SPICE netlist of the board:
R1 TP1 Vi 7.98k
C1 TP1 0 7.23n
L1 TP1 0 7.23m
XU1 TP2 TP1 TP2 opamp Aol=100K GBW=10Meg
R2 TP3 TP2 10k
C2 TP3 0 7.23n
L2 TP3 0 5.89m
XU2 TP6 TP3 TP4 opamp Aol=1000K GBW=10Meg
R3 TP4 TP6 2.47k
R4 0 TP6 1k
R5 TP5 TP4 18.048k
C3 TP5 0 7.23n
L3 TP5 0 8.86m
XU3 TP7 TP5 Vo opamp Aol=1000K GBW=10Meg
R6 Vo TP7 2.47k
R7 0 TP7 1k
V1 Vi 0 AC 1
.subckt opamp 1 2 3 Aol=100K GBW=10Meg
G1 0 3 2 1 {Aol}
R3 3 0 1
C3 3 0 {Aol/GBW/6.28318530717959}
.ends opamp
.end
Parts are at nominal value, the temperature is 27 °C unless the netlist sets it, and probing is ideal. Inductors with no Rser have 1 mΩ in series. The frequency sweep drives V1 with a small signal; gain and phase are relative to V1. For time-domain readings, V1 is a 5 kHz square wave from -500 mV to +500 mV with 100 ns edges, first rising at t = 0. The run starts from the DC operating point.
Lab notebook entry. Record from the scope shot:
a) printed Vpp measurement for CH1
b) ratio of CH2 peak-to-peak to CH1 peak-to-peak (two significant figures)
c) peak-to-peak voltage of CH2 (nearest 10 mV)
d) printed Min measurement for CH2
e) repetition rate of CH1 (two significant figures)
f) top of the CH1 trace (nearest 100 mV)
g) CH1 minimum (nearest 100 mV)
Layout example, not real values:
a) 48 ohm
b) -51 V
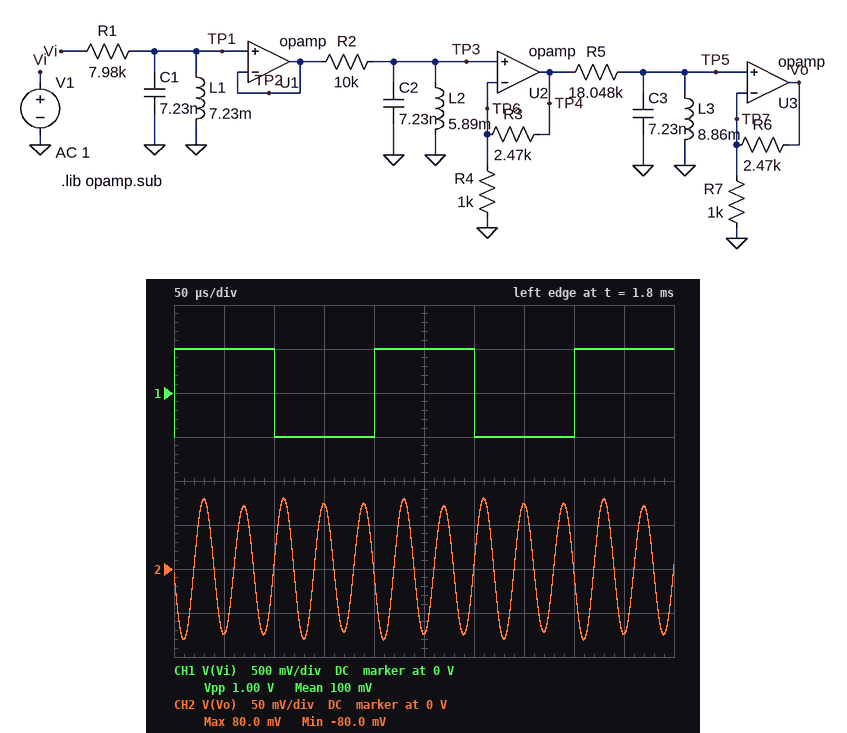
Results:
a) 1.00 V
b) 0.16
c) 160 mV
d) -80.0 mV
e) 5.0 kHz
f) 500 mV
g) -500 mV
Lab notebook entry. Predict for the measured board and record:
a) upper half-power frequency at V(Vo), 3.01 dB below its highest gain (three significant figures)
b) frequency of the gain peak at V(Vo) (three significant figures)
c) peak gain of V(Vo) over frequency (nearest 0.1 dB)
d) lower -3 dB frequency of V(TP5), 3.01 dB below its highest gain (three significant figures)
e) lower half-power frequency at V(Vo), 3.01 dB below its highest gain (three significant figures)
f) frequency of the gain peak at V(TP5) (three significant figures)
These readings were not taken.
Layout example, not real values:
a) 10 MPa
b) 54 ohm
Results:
a) 24.1 kHz
b) 20.2 kHz
c) 3.3 dB
d) 19.6 kHz
e) 19.6 kHz
f) 20.2 kHz
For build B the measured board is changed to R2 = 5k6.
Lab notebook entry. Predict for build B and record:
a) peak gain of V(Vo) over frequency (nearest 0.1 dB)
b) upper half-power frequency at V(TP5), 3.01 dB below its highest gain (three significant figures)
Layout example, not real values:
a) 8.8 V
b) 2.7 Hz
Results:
a) 7.9 dB
b) 22.8 kHz
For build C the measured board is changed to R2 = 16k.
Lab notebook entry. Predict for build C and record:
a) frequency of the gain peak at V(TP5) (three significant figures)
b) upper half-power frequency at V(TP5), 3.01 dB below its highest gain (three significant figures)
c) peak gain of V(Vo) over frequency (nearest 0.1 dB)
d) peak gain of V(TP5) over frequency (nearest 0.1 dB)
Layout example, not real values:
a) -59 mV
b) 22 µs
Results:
a) 24.1 kHz
b) 24.7 kHz
c) -0.1 dB
d) -10.9 dB
